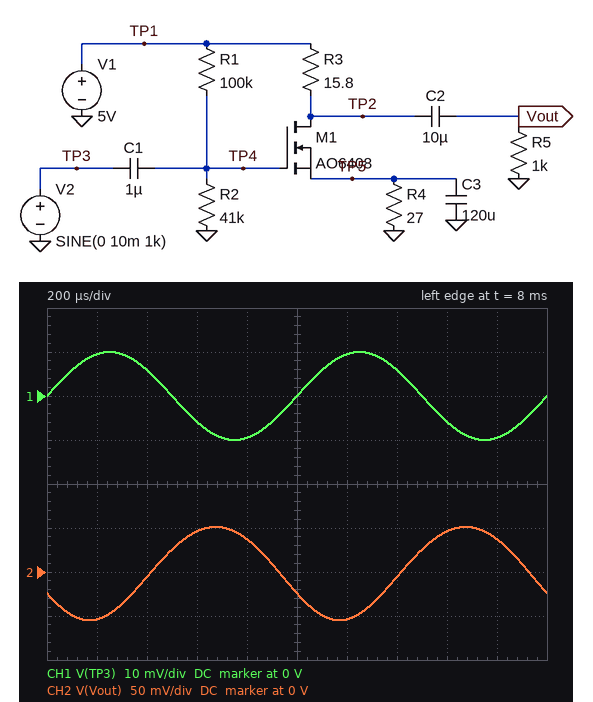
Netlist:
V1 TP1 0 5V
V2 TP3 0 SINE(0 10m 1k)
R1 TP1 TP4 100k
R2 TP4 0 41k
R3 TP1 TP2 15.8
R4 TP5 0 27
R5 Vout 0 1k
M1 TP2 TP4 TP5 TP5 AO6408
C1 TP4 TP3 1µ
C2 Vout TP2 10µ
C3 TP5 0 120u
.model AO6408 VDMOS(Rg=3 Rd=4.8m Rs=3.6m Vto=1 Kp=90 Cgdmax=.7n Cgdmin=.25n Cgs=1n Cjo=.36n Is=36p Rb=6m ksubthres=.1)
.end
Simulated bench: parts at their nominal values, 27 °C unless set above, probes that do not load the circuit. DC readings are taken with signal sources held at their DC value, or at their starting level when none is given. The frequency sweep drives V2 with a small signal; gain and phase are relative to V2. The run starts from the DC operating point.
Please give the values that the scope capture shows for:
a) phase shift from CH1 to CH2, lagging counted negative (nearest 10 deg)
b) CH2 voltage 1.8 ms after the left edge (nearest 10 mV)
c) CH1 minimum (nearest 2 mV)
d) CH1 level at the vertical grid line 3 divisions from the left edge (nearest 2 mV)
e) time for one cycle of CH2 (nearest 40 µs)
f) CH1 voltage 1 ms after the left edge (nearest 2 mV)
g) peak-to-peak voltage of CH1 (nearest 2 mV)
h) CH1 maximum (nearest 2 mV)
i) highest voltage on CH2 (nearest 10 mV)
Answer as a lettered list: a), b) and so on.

a) -150 deg
b) 40 mV
c) -10 mV
d) -6 mV
e) 1.00 ms
f) 0 V
g) 20 mV
h) 10 mV
i) 50 mV
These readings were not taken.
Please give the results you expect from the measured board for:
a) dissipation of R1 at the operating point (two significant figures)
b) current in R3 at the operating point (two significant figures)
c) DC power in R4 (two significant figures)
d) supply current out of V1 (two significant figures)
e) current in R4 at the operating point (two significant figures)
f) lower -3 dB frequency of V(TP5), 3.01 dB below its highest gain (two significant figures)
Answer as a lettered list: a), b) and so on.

a) 130 µW
b) 22 mA
c) 13 mW
d) 22 mA
e) 22 mA
f) 5.4 Hz
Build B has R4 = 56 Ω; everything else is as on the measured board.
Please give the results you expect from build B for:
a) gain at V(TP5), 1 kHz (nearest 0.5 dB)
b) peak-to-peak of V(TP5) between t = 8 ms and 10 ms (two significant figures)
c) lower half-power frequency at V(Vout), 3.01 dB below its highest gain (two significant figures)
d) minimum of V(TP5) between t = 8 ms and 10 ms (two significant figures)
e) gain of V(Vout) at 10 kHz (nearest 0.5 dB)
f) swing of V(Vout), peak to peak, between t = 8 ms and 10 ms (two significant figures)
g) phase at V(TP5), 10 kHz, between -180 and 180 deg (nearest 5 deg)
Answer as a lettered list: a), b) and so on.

a) -11.5 dB
b) 5.3 mV
c) 300 Hz
d) 630 mV
e) 10.0 dB
f) 62 mV
g) -90 deg
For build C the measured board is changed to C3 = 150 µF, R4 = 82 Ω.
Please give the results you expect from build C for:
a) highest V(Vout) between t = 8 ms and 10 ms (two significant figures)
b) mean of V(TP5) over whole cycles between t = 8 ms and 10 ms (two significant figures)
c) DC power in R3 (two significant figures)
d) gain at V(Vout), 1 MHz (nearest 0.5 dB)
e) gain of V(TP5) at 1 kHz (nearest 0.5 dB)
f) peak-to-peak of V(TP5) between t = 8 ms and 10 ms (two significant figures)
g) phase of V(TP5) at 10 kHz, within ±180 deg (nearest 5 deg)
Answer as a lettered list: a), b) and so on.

a) 22 mV
b) 650 mV
c) 990 µW
d) 7.0 dB
e) -16.0 dB
f) 3.1 mV
g) -90 deg
